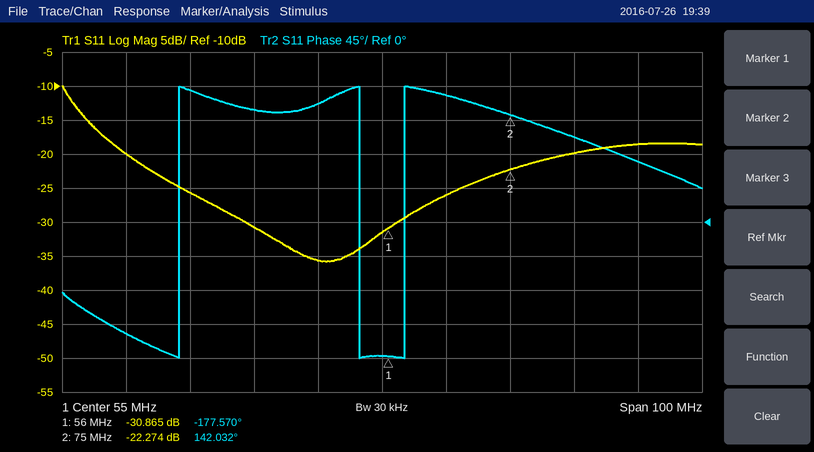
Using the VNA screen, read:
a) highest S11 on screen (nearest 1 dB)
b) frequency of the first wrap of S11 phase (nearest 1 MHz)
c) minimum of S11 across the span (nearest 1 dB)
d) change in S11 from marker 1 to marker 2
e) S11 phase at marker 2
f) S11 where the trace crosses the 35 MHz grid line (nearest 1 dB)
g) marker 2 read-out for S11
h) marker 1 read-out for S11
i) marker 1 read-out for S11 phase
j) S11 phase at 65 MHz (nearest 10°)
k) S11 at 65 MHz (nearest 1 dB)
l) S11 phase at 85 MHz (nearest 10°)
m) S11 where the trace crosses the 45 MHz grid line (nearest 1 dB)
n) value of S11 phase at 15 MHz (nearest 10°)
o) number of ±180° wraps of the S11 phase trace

-10 dB
23 MHz
-36 dB
8.591 dB
142.032°
-31 dB
-22.274 dB
-30.865 dB
-177.570°
170°
-26 dB
110°
-36 dB
-150°
3
